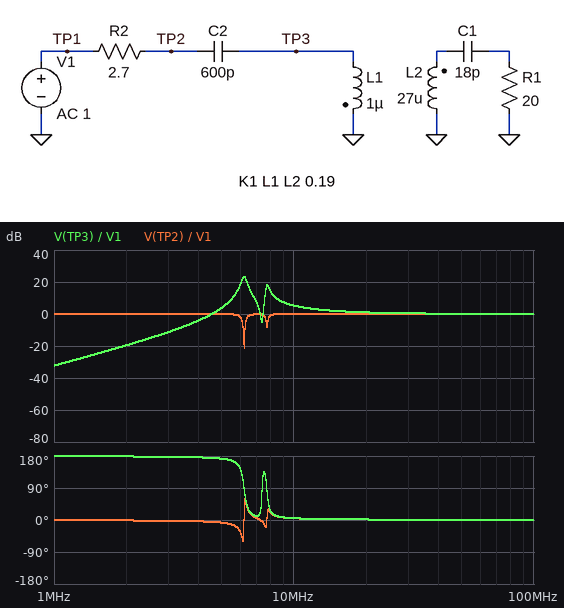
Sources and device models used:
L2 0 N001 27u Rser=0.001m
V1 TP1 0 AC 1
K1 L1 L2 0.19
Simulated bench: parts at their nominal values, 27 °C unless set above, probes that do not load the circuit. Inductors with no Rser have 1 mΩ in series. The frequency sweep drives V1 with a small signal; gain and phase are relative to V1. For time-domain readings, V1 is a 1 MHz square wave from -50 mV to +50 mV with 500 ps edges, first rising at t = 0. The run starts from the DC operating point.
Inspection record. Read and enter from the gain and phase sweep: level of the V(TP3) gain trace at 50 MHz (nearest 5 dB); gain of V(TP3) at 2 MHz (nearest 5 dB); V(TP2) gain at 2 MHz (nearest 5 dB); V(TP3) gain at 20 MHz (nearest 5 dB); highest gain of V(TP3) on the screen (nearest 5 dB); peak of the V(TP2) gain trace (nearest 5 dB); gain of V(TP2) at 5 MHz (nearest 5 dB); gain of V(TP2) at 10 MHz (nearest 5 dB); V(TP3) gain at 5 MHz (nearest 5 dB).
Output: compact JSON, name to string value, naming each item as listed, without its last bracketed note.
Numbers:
{"level of the V(TP3) gain trace at 50 MHz": "0 dB", "gain of V(TP3) at 2 MHz": "-20 dB", "V(TP2) gain at 2 MHz": "0 dB", "V(TP3) gain at 20 MHz": "0 dB", "highest gain of V(TP3) on the screen": "25 dB", "peak of the V(TP2) gain trace": "0 dB", "gain of V(TP2) at 5 MHz": "0 dB", "gain of V(TP2) at 10 MHz": "0 dB", "V(TP3) gain at 5 MHz": "5 dB"}
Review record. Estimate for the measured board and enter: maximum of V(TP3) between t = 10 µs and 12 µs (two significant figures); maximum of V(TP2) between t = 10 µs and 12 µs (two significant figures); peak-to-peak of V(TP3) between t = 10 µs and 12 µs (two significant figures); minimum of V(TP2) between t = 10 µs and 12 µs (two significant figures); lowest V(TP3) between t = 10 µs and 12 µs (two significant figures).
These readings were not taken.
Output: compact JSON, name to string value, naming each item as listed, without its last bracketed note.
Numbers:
{"maximum of V(TP3) between t = 10 µs and 12 µs": "61 mV", "maximum of V(TP2) between t = 10 µs and 12 µs": "53 mV", "peak-to-peak of V(TP3) between t = 10 µs and 12 µs": "120 mV", "minimum of V(TP2) between t = 10 µs and 12 µs": "-53 mV", "lowest V(TP3) between t = 10 µs and 12 µs": "-61 mV"}
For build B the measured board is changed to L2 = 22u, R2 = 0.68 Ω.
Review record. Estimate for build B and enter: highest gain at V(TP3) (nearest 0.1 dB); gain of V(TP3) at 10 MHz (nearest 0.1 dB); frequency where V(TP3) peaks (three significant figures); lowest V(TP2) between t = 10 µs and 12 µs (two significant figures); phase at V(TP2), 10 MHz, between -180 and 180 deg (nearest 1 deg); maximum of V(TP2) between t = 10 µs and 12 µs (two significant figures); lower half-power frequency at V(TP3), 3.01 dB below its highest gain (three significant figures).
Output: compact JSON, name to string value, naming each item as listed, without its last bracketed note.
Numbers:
{"highest gain at V(TP3)": "34.7 dB", "gain of V(TP3) at 10 MHz": "5.5 dB", "frequency where V(TP3) peaks": "6.31 MHz", "lowest V(TP2) between t = 10 µs and 12 µs": "-51 mV", "phase at V(TP2), 10 MHz, between -180 and 180 deg": "1 deg", "maximum of V(TP2) between t = 10 µs and 12 µs": "51 mV", "lower half-power frequency at V(TP3), 3.01 dB below its highest gain": "6.26 MHz"}
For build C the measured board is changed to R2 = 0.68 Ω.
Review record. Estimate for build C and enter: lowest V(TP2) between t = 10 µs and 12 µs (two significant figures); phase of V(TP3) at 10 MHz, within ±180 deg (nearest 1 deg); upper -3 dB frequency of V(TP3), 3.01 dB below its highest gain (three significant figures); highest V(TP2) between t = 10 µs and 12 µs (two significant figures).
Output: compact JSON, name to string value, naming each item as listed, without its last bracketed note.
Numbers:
{"lowest V(TP2) between t = 10 µs and 12 µs": "-51 mV", "phase of V(TP3) at 10 MHz, within ±180 deg": "1 deg", "upper -3 dB frequency of V(TP3), 3.01 dB below its highest gain": "6.24 MHz", "highest V(TP2) between t = 10 µs and 12 µs": "51 mV"}
